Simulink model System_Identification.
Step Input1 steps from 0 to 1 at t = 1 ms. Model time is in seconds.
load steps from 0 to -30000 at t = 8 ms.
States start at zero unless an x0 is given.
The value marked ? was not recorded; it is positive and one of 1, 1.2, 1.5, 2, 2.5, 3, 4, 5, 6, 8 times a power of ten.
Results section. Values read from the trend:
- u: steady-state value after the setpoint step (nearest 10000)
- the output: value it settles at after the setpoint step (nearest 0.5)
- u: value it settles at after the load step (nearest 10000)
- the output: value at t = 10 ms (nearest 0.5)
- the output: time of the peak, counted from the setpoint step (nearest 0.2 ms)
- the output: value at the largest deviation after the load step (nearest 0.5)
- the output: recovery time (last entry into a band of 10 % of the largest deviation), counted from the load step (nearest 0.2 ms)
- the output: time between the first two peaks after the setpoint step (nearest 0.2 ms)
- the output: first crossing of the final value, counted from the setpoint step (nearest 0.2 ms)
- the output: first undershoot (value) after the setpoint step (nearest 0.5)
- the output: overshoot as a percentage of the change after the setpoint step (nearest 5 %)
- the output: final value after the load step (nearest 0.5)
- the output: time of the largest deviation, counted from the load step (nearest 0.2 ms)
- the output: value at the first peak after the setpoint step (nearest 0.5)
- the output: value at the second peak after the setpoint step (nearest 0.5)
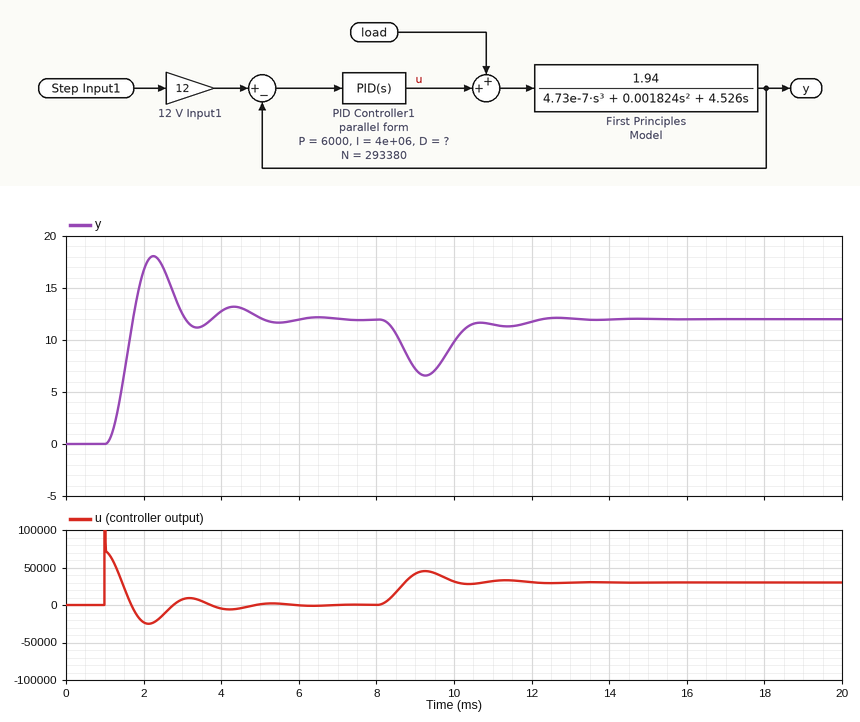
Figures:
0
12.0
30000
10.0
1.2 ms
6.5
3.8 ms
2.0 ms
0.8 ms
11.0
50 %
12.0
1.2 ms
18.0
13.0
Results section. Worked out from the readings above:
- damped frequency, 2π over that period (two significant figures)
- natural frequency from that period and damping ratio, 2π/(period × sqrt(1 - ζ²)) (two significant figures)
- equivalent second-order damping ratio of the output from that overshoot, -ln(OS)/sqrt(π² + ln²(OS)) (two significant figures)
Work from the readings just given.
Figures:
3.1 rad/ms
3.2 rad/ms
0.22
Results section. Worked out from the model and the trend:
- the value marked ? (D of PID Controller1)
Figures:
1.2
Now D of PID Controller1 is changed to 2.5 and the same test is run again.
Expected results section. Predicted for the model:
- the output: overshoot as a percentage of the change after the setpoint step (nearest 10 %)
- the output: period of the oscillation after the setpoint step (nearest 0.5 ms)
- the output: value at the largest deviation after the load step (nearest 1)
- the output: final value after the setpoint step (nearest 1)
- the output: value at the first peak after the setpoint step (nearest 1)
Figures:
30 %
1.5 ms
8
12
15
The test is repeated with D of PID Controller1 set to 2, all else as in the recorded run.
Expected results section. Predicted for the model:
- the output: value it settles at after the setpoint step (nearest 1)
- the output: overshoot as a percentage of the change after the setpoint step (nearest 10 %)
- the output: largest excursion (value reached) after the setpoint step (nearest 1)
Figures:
12
30 %
16
